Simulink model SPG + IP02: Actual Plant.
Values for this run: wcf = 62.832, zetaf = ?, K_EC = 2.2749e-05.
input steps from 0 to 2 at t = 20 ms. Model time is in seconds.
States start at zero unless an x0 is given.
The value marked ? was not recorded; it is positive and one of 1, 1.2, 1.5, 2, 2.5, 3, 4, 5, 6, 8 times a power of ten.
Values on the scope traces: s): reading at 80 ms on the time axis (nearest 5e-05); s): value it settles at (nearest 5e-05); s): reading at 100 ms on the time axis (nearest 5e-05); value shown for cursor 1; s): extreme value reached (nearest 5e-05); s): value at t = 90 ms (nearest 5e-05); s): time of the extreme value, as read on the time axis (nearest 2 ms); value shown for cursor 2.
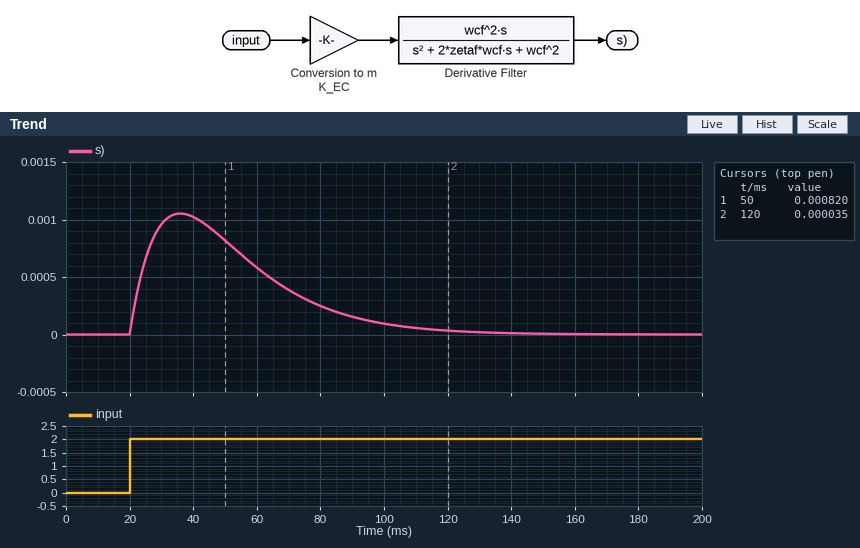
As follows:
0.00025
0.00000
0.00010
0.000820
0.00105
0.00015
36 ms
0.000035
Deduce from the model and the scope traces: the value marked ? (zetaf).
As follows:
1
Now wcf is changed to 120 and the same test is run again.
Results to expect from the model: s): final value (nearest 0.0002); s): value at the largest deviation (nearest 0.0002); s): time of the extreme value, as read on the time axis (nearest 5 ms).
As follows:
0.0000
0.0020
30 ms
